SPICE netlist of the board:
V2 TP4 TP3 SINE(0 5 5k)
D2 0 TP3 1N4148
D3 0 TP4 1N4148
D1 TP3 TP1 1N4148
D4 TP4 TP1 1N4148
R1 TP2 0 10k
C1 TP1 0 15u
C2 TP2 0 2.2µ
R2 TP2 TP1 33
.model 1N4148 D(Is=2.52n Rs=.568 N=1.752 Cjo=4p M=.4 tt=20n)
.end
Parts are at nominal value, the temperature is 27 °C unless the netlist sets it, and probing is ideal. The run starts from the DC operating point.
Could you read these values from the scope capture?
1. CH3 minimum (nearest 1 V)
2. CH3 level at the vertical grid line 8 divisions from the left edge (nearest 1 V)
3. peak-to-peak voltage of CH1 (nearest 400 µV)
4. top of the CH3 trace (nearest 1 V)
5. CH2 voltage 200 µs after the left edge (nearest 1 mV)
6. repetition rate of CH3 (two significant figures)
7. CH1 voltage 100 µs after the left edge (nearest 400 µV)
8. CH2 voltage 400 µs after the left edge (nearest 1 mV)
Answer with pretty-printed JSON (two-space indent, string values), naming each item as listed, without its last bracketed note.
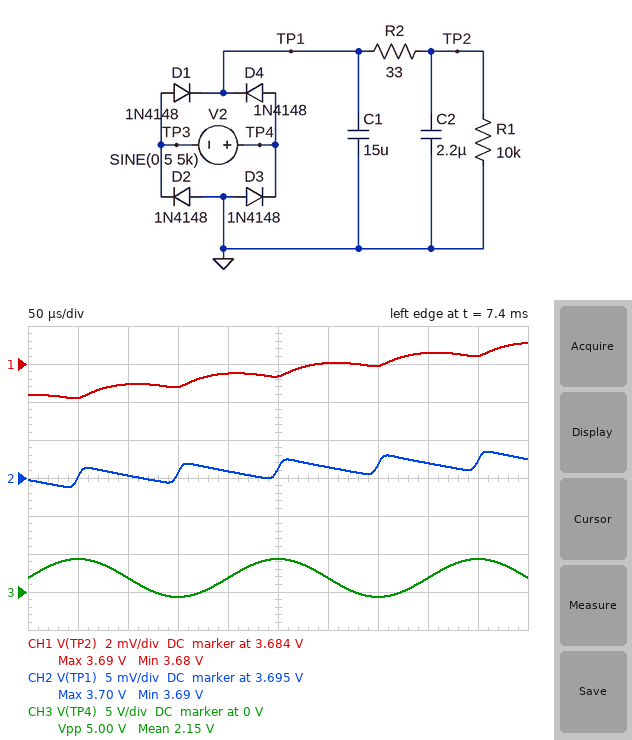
{
  "CH3 minimum": "-1 V",
  "CH3 level at the vertical grid line 8 divisions from the left edge": "2 V",
  "peak-to-peak voltage of CH1": "2.8 mV",
  "top of the CH3 trace": "4 V",
  "CH2 voltage 200 µs after the left edge": "3.696 V",
  "repetition rate of CH3": "5.0 kHz",
  "CH1 voltage 100 µs after the left edge": "3.6828 V",
  "CH2 voltage 400 µs after the left edge": "3.697 V"
}
